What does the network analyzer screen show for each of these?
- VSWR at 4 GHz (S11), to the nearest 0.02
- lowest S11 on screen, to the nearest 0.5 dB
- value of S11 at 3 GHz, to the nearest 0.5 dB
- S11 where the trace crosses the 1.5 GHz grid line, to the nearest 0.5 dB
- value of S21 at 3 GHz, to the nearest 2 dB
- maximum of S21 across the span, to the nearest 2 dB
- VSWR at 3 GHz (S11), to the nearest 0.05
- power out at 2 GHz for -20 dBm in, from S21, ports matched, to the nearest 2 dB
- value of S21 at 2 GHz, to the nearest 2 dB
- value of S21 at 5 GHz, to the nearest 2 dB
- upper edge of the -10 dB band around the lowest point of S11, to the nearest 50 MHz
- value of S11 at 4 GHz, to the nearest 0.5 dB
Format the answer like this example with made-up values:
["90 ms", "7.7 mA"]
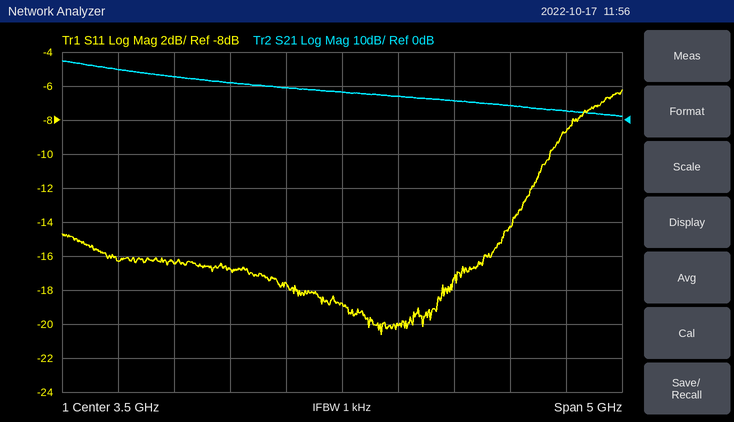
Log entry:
["1.22", "-20.5 dB", "-17.5 dB", "-16.5 dB", "10 dB", "18 dB", "1.30", "-8 dBm", "12 dB", "4 dB", "5.35 GHz", "-20.0 dB"]
